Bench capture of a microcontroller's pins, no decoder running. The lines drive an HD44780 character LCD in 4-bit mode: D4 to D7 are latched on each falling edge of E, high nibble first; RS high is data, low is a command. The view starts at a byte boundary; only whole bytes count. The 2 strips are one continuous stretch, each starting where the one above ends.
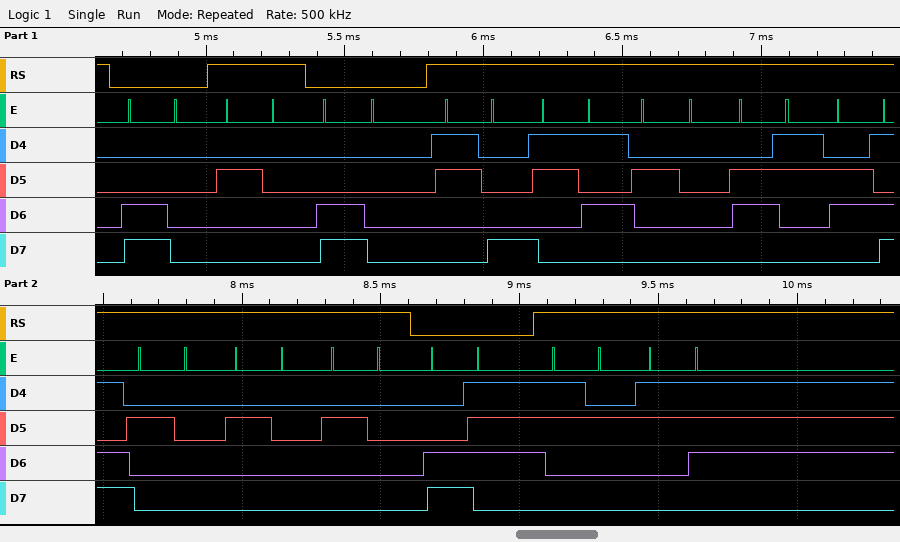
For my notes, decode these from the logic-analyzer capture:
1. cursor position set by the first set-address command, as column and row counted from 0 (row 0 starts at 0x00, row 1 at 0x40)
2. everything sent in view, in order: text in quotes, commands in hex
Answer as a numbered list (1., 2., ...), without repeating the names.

1. column 0, row 1
2. 0xC0 " " 0xC0 "85 cm   " 0xC7 "27"
